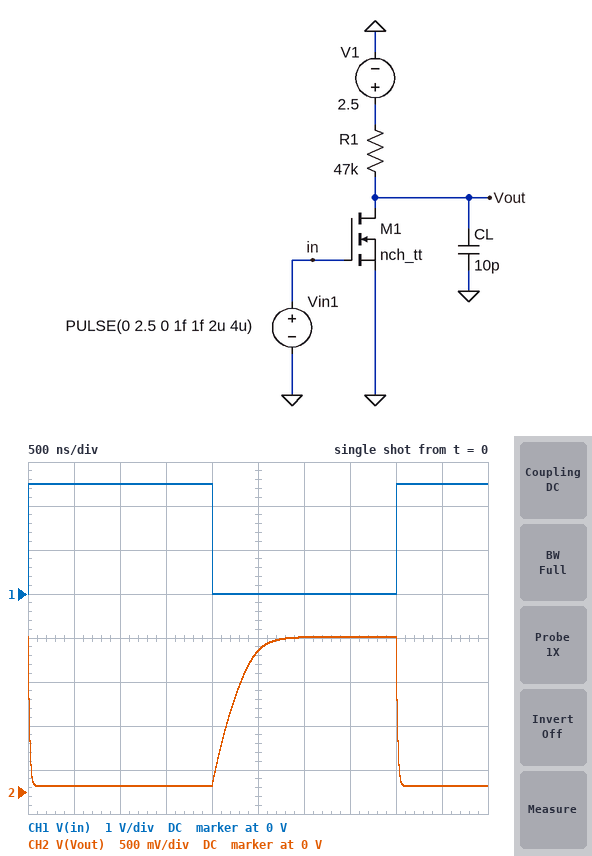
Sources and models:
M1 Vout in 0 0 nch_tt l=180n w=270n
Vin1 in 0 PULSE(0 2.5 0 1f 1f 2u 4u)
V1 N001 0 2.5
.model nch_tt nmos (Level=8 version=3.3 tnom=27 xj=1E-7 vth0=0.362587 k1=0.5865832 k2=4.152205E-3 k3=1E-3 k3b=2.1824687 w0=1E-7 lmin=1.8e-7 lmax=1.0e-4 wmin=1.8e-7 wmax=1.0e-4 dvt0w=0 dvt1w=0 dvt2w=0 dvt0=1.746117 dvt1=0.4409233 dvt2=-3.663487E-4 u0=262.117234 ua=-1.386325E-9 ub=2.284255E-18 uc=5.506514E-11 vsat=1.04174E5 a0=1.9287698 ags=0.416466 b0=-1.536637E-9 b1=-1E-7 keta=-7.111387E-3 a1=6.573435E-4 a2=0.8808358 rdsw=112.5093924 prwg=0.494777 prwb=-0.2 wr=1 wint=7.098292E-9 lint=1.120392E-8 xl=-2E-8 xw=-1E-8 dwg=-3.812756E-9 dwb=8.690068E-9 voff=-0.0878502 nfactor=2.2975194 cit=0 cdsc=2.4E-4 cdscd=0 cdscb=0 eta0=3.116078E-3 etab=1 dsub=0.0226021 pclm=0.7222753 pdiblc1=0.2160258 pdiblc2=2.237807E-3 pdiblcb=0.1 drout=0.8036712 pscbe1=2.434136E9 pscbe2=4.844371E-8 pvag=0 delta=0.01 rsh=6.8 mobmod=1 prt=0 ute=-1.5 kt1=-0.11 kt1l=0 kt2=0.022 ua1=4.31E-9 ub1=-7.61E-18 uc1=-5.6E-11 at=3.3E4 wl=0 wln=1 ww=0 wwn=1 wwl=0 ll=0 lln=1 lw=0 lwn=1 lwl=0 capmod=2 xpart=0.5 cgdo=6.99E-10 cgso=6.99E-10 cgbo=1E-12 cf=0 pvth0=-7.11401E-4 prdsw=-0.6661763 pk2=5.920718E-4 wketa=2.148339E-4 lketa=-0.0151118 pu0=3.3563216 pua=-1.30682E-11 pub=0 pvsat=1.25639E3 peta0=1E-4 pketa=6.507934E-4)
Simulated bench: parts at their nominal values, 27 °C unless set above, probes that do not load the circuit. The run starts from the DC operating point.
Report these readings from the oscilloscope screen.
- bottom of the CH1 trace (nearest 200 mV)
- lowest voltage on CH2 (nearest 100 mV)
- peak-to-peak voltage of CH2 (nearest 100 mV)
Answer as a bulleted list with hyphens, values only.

- 0 V
- 100 mV
- 1.7 V
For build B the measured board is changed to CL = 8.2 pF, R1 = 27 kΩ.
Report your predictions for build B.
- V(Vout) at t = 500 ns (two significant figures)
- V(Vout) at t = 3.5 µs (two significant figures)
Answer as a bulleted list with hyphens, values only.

- 120 mV
- 1.9 V
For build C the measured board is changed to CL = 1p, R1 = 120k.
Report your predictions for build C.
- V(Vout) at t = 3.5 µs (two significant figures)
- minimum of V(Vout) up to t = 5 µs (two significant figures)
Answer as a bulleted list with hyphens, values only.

- 1.6 V
- 26 mV
